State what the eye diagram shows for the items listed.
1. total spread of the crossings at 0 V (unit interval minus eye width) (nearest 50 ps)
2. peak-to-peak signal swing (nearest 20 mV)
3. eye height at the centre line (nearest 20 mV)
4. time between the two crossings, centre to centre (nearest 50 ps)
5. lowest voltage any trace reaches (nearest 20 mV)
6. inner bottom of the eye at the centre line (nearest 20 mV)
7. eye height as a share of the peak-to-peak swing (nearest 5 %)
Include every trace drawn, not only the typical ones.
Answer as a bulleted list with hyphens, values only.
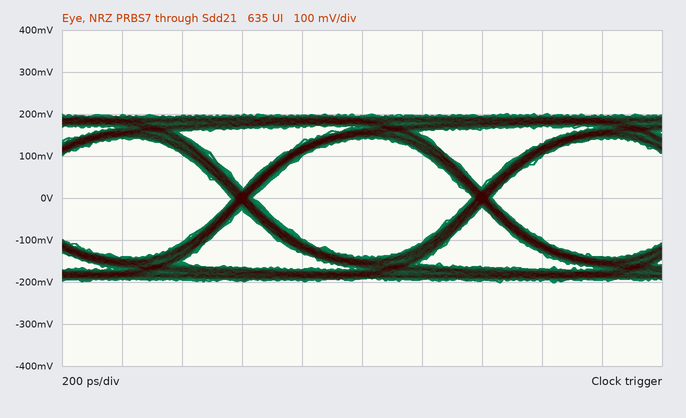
- 50 ps
- 400 mV
- 280 mV
- 800 ps
- -200 mV
- -140 mV
- 70 %
